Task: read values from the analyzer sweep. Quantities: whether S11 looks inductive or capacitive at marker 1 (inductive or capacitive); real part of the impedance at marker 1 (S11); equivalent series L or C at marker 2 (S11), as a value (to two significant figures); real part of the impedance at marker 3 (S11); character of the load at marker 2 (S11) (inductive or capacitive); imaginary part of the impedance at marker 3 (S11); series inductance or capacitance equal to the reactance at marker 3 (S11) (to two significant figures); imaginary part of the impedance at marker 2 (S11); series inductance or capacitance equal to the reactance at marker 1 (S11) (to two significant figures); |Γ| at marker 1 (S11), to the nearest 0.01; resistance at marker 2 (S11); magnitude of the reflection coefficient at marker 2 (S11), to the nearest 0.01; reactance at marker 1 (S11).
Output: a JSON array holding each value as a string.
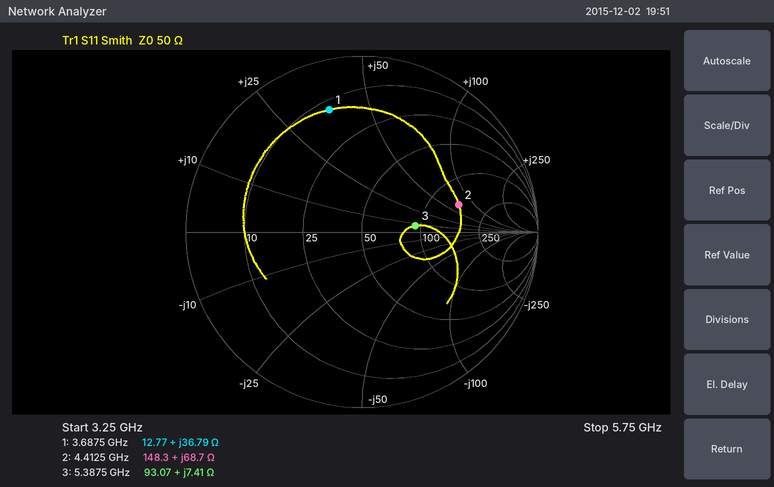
["inductive", "12.77 Ω", "2.5 nH", "93.07 Ω", "inductive", "+7.41 Ω", "220 pH", "+68.7 Ω", "1.6 nH", "0.72", "148.3 Ω", "0.57", "+36.79 Ω"]
